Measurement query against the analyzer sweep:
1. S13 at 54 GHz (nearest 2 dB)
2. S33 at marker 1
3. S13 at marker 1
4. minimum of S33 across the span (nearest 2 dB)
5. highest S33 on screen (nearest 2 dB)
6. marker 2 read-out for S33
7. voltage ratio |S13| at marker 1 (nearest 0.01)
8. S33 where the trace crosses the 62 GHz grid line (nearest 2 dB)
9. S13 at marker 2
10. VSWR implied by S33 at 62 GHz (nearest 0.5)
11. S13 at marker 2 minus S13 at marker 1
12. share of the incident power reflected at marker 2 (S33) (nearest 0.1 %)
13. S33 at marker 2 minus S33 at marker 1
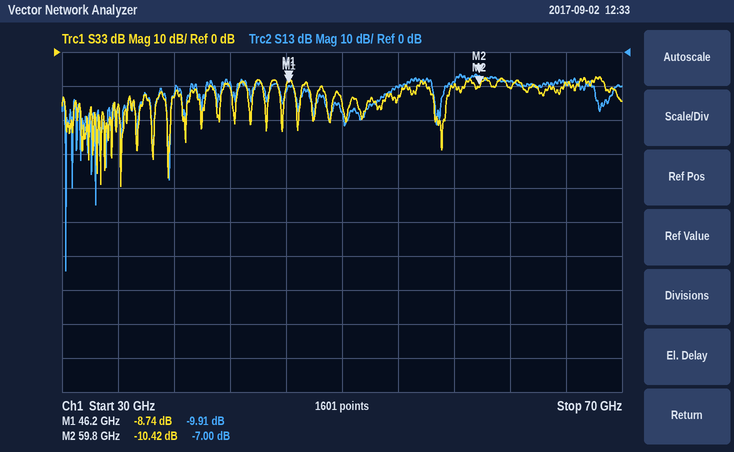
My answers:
-10 dB
-8.74 dB
-9.91 dB
-40 dB
-8 dB
-10.42 dB
0.32
-10 dB
-7.00 dB
2.0
2.91 dB
9.1 %
-1.68 dB
